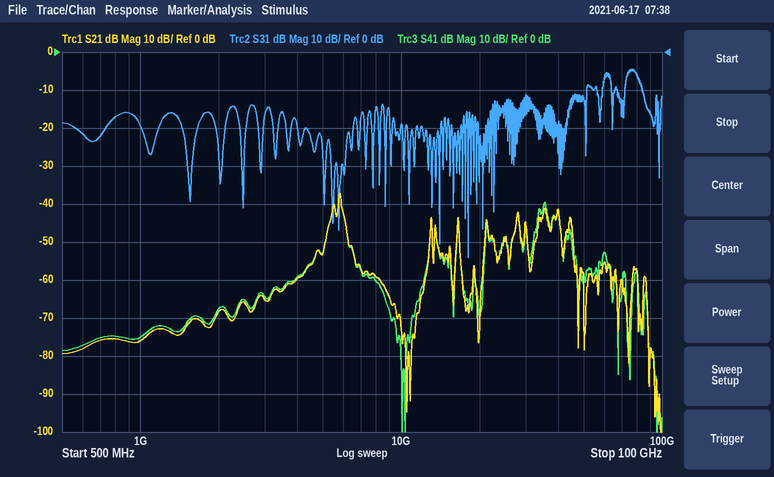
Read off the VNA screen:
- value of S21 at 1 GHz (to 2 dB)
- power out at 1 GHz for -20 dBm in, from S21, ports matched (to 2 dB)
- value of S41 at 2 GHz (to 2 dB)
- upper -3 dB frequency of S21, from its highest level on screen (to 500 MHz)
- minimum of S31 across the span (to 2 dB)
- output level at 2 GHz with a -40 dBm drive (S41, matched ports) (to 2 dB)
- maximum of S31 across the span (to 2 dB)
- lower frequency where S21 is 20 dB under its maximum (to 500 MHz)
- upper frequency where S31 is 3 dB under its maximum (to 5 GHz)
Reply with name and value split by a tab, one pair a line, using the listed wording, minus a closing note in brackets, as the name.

value of S21 at 1 GHz	-76 dB
power out at 1 GHz for -20 dBm in, from S21, ports matched	-96 dBm
value of S41 at 2 GHz	-68 dB
upper -3 dB frequency of S21, from its highest level on screen	6.0 GHz
minimum of S31 across the span	-54 dB
output level at 2 GHz with a -40 dBm drive (S41, matched ports)	-108 dBm
maximum of S31 across the span	-4 dB
lower frequency where S21 is 20 dB under its maximum	4.5 GHz
upper frequency where S31 is 3 dB under its maximum	80 GHz
